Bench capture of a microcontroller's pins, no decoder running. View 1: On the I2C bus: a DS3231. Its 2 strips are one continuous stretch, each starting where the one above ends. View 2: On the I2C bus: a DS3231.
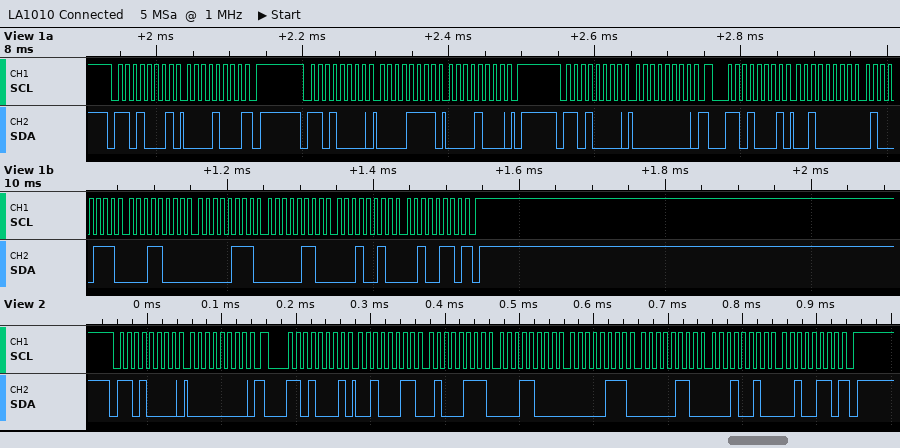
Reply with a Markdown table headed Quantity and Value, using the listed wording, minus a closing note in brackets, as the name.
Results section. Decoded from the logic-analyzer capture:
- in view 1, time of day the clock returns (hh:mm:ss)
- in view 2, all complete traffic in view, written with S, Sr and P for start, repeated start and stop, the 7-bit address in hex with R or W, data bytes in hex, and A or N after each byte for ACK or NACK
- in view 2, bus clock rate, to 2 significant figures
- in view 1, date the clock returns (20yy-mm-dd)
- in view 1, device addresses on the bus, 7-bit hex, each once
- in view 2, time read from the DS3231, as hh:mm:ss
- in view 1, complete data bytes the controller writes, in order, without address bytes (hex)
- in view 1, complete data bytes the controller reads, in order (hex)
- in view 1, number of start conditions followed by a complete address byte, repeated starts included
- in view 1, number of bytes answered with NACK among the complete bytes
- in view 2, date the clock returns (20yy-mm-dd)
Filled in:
| Quantity | Value |
|---|---|
| in view 1, time of day the clock returns | 18:47:20 |
| in view 2, all complete traffic in view, written with S, Sr and P for start, repeated start and stop, the 7-bit address in hex with R or W, data bytes in hex, and A or N after each byte for ACK or NACK | S 68W A 00 A Sr 68R A 23 A 47 A 18 A 07 A 06 A 12 A 26 N P |
| in view 2, bus clock rate, to 2 significant figures | 100 kHz |
| in view 1, date the clock returns | 2026-12-06 |
| in view 1, device addresses on the bus, 7-bit hex, each once | 0x68 |
| in view 2, time read from the DS3231, as hh:mm:ss | 18:47:23 |
| in view 1, complete data bytes the controller writes, in order, without address bytes | 0F 08 00 |
| in view 1, complete data bytes the controller reads, in order | 08 20 47 18 07 06 12 26 |
| in view 1, number of start conditions followed by a complete address byte, repeated starts included | 4 |
| in view 1, number of bytes answered with NACK among the complete bytes | 2 |
| in view 2, date the clock returns | 2026-12-06 |
